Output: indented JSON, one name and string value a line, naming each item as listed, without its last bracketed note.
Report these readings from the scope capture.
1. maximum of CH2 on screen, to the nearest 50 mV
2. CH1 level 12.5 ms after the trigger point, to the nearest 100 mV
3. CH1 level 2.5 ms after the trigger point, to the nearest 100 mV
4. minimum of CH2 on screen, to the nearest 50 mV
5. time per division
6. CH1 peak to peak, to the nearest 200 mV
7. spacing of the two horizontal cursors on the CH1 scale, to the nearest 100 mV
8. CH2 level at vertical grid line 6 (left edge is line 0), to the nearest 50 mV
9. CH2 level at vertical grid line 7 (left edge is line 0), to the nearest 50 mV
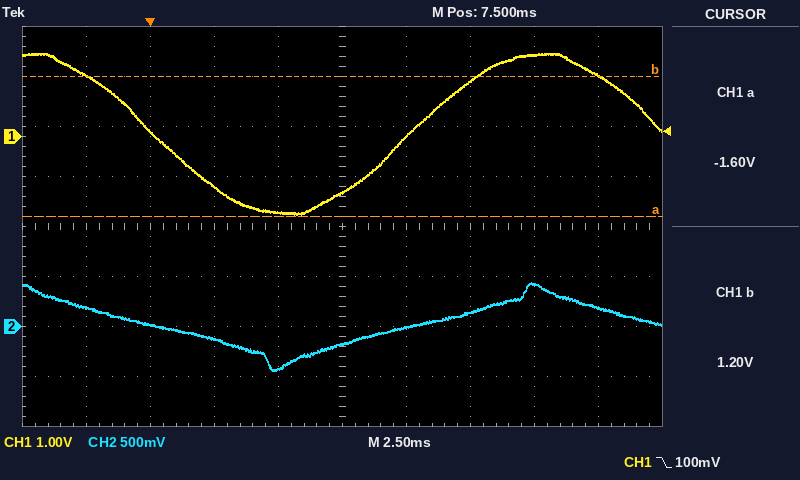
{
  "maximum of CH2 on screen, to the nearest 50 mV": "450 mV",
  "CH1 level 12.5 ms after the trigger point, to the nearest 100 mV": "1.1 V",
  "CH1 level 2.5 ms after the trigger point, to the nearest 100 mV": "-1.0 V",
  "minimum of CH2 on screen, to the nearest 50 mV": "-450 mV",
  "time per division": "2.5 ms",
  "CH1 peak to peak, to the nearest 200 mV": "3.2 V",
  "spacing of the two horizontal cursors on the CH1 scale, to the nearest 100 mV": "2.8 V",
  "CH2 level at vertical grid line 6 (left edge is line 0), to the nearest 50 mV": "0 mV",
  "CH2 level at vertical grid line 7 (left edge is line 0), to the nearest 50 mV": "150 mV"
}
